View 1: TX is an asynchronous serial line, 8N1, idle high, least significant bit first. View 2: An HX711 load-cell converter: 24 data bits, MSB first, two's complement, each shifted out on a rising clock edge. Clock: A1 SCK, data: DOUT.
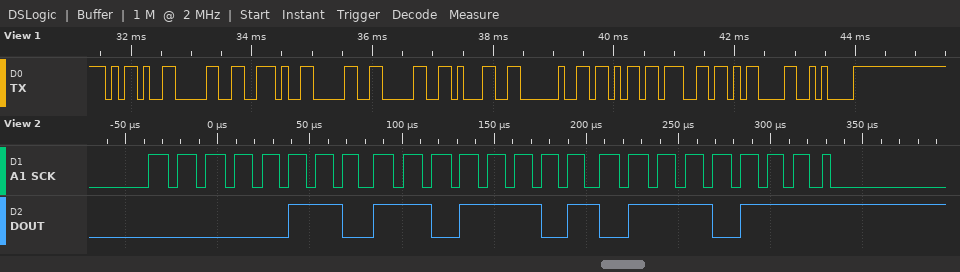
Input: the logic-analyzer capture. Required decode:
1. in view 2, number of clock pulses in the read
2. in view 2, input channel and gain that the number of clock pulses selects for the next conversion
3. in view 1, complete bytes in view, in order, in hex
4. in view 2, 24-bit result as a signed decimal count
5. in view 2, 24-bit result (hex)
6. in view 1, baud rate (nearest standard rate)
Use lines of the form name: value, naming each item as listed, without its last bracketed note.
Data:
in view 2, number of clock pulses in the read: 25
in view 2, input channel and gain that the number of clock pulses selects for the next conversion: channel A, gain 128
in view 1, complete bytes in view, in order, in hex: 2D 30 2E 30 30 31 20 6B 67 0D 0A
in view 2, 24-bit result as a signed decimal count: 449911
in view 2, 24-bit result: 0x06DD77
in view 1, baud rate: 9600 baud
